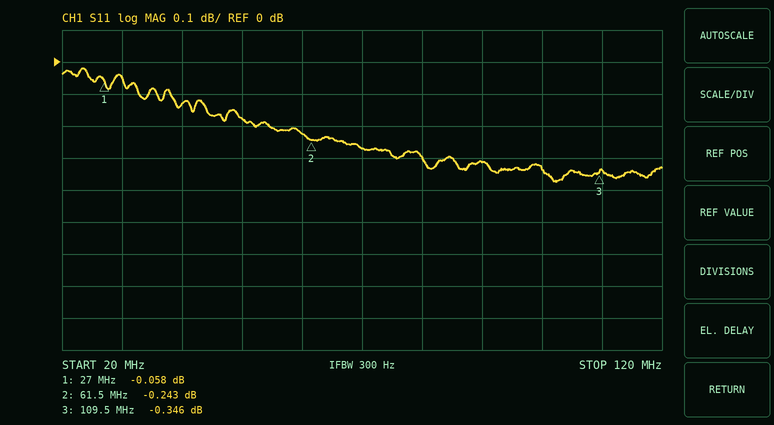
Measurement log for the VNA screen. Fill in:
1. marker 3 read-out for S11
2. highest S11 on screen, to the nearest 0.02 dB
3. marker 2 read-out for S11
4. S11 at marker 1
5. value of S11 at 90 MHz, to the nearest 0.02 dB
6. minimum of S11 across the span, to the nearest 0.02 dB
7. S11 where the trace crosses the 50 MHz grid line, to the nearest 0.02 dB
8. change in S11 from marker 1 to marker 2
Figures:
-0.346 dB
-0.02 dB
-0.243 dB
-0.058 dB
-0.32 dB
-0.38 dB
-0.18 dB
-0.185 dB
